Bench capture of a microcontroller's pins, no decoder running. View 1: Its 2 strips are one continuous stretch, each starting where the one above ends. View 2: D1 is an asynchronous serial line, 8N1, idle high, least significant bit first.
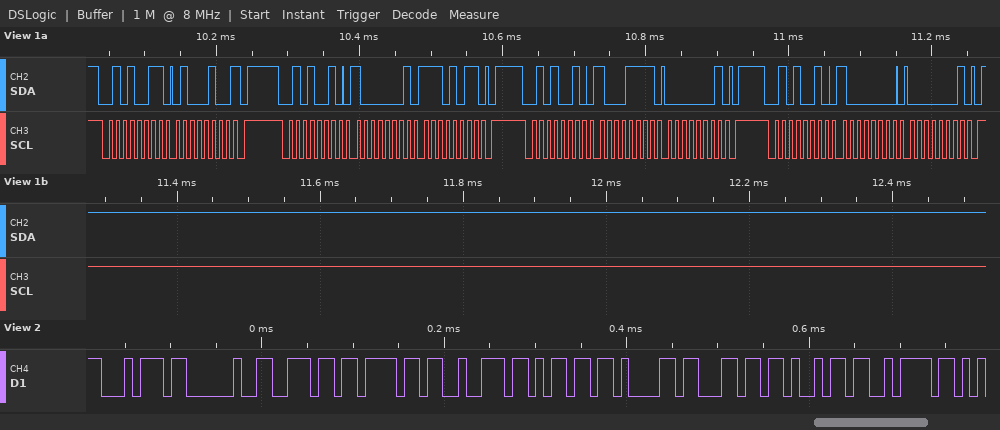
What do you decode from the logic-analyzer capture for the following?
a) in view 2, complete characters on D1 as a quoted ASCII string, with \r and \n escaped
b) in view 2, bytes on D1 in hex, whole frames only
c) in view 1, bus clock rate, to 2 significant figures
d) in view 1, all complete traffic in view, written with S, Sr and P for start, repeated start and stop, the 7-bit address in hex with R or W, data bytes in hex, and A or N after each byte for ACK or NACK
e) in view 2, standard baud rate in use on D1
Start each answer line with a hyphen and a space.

- "t normaliz"
- 74 20 6E 6F 72 6D 61 6C 69 7A
- 100 kHz
- S 29R A 44 N P S 29W A 81 A EB A P S 29W A 8F A 01 A P S 29W A 80 A 01 A P
- 115200 baud
